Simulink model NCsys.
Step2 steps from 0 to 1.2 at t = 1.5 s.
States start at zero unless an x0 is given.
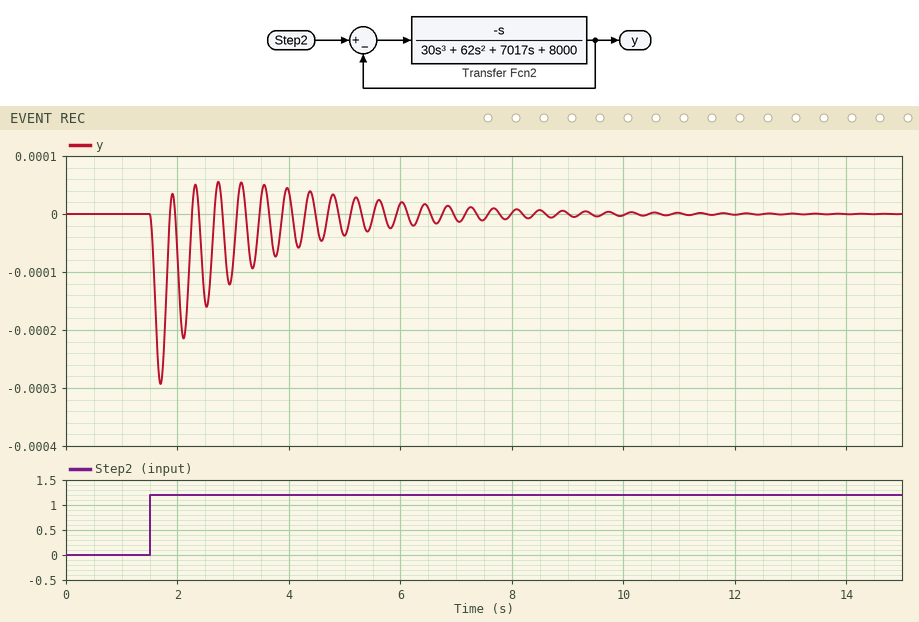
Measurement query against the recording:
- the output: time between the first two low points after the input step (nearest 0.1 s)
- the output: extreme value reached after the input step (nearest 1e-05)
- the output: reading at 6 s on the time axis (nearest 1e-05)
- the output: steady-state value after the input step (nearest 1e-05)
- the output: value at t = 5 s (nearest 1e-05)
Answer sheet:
0.4 s
-0.00029
0.00002
0.00000
-0.00004
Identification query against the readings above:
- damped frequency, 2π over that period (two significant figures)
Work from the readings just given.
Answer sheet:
16 rad/s
